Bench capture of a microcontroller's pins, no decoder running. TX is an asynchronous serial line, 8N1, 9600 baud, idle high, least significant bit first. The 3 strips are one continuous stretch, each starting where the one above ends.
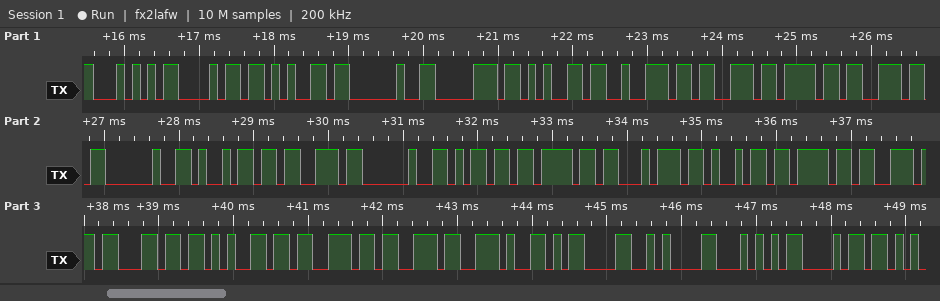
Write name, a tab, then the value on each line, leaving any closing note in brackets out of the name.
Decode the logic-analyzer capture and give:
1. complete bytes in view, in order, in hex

complete bytes in view, in order, in hex	0x54 0x68 0x65 0x20 0x70 0x65 0x72 0x73 0x6F 0x6E 0x20 0x69 0x73 0x20 0x6D 0x6F 0x74 0x69 0x6F 0x6E 0x6C 0x65 0x73 0x73 0x2E 0x0D 0x0A 0x54 0x68
